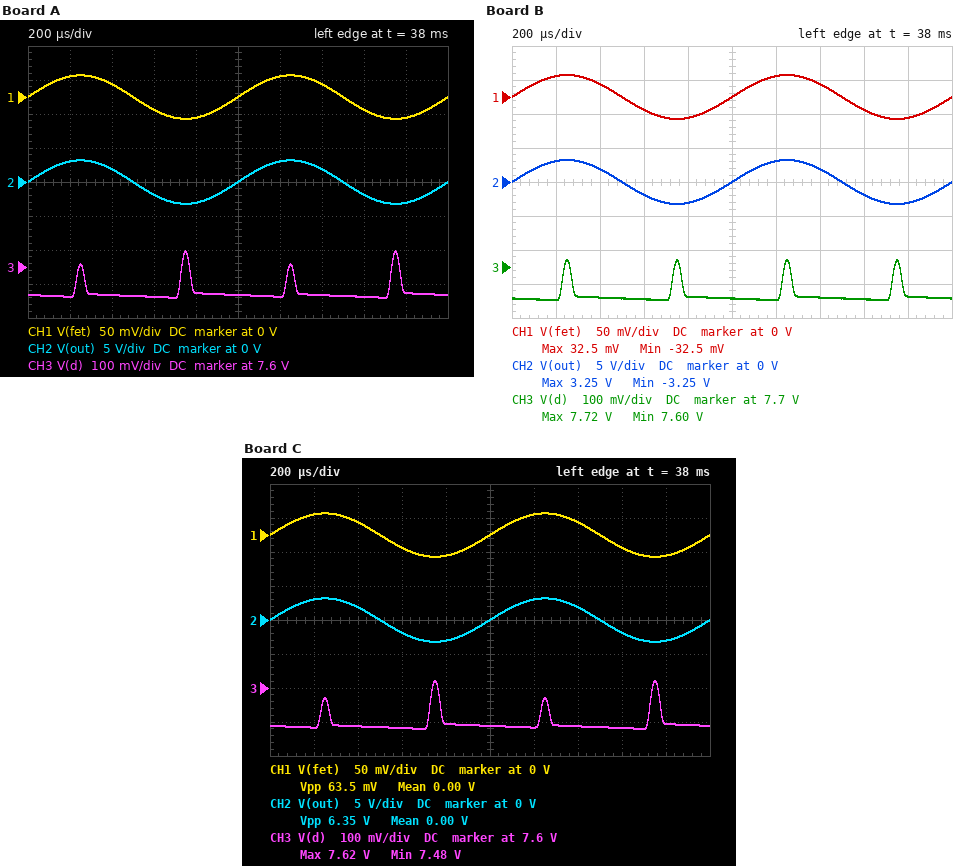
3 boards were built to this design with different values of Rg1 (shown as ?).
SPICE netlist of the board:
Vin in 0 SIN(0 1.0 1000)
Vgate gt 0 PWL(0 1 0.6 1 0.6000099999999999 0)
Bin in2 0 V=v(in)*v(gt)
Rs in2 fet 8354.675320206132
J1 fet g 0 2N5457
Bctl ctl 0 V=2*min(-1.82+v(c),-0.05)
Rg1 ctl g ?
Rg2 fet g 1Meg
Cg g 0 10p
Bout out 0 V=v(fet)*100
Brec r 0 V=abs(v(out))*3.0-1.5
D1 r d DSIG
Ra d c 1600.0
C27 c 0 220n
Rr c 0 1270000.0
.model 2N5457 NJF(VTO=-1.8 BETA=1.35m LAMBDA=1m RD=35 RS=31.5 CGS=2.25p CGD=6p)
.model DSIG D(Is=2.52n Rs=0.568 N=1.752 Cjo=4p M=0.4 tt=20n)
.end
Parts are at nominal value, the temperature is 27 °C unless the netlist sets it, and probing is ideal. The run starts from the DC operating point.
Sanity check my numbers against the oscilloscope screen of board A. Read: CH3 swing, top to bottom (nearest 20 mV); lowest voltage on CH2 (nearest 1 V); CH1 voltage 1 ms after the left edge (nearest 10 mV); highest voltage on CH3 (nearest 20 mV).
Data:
140 mV
-3 V
0 V
7.64 V
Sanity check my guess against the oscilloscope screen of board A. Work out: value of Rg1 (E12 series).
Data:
2.2 MΩ
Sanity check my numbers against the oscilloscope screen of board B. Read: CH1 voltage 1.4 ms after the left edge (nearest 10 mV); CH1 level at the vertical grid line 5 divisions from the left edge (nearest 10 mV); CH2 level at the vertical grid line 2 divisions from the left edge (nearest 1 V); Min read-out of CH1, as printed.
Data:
20 mV
0 V
2 V
-32.5 mV
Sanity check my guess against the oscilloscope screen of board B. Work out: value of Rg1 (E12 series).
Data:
820 kΩ
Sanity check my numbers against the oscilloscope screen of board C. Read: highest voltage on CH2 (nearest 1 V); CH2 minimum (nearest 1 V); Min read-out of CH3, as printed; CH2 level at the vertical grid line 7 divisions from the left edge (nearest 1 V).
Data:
3 V
-3 V
7.48 V
2 V
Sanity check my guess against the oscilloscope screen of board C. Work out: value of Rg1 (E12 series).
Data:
3.3 MΩ
